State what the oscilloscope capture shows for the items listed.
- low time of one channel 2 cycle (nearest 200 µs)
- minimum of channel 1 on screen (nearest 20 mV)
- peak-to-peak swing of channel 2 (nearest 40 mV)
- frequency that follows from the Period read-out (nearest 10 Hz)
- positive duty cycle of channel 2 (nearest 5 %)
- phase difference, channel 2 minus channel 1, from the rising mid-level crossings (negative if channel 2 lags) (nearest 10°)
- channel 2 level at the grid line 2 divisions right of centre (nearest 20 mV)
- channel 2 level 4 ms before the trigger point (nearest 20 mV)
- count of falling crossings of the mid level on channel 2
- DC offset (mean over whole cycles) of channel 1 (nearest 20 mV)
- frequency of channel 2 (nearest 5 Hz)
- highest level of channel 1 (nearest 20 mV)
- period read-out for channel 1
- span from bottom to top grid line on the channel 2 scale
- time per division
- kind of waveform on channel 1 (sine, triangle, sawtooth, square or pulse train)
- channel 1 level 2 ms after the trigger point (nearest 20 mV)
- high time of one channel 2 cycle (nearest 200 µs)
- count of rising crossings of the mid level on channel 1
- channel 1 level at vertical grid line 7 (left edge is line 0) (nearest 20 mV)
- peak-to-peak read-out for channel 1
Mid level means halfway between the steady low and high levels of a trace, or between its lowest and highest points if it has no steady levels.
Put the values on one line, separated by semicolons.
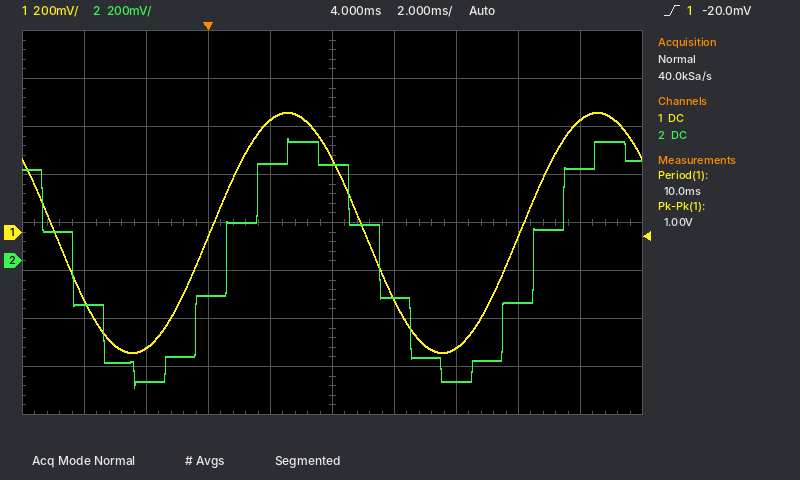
5.0 ms; -500 mV; 1.04 V; 100 Hz; 50 %; -20°; -500 mV; -180 mV; 2; 0 mV; 100 Hz; 500 mV; 10.0 ms; 1.6 V; 2 ms; sine; 460 mV; 5.0 ms; 2; -480 mV; 1.00 V
